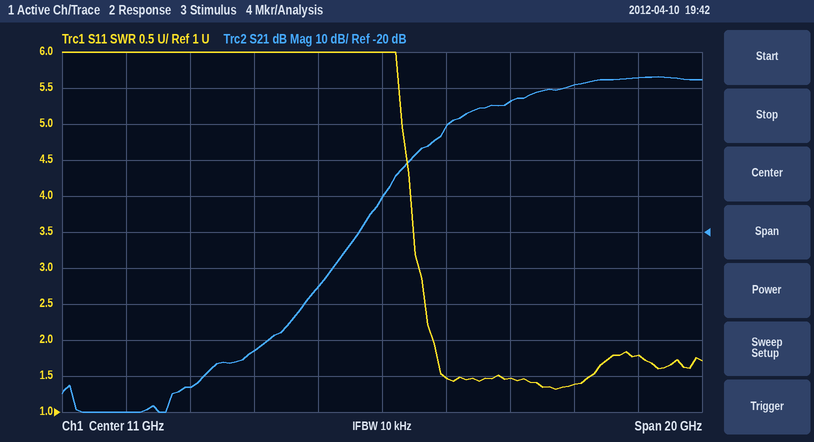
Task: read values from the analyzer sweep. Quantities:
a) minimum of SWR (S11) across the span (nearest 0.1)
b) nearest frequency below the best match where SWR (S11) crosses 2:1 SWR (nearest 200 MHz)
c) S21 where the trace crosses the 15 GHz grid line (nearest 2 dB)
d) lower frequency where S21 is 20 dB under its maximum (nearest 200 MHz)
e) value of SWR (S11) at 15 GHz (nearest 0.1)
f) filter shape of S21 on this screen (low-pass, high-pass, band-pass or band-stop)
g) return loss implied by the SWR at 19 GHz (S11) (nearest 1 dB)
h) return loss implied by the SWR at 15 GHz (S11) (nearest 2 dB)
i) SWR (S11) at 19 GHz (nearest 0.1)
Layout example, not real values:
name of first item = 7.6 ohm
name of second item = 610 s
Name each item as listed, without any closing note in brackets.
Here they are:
minimum of SWR (S11) across the span = 1.3
nearest frequency below the best match where SWR (S11) crosses 2:1 SWR = 12.6 GHz
S21 where the trace crosses the 15 GHz grid line = 16 dB
lower frequency where S21 is 20 dB under its maximum = 12.2 GHz
value of SWR (S11) at 15 GHz = 1.5
filter shape of S21 on this screen = high-pass
return loss implied by the SWR at 19 GHz (S11) = 11 dB
return loss implied by the SWR at 15 GHz (S11) = 14 dB
SWR (S11) at 19 GHz = 1.8
